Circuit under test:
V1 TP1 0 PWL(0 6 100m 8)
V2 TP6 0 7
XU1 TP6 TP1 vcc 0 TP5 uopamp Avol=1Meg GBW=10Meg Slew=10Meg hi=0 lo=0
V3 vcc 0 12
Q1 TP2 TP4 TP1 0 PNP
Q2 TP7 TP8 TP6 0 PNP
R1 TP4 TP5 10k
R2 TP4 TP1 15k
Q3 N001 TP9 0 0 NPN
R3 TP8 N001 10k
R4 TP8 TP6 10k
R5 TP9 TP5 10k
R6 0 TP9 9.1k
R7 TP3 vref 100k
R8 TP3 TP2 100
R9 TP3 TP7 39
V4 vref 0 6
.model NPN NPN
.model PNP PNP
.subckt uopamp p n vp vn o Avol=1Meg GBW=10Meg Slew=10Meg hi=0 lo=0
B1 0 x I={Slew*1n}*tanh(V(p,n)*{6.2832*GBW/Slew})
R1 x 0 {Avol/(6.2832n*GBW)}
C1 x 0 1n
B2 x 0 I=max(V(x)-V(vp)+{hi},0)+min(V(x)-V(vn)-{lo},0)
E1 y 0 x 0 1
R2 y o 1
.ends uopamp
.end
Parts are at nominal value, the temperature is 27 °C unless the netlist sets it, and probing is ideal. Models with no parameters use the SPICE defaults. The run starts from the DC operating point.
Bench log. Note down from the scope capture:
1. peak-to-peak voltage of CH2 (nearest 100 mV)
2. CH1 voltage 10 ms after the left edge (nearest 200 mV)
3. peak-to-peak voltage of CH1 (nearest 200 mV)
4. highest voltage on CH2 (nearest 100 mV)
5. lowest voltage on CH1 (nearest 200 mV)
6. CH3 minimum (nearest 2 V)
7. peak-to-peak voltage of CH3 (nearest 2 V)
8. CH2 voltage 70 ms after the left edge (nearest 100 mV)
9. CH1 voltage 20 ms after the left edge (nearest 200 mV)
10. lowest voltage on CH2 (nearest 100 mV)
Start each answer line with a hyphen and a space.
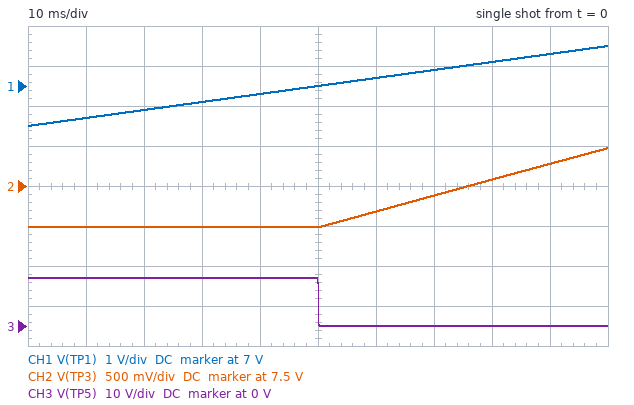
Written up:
- 1.0 V
- 6.2 V
- 2.0 V
- 8.0 V
- 6.0 V
- 0 V
- 12 V
- 7.4 V
- 6.4 V
- 7.0 V
